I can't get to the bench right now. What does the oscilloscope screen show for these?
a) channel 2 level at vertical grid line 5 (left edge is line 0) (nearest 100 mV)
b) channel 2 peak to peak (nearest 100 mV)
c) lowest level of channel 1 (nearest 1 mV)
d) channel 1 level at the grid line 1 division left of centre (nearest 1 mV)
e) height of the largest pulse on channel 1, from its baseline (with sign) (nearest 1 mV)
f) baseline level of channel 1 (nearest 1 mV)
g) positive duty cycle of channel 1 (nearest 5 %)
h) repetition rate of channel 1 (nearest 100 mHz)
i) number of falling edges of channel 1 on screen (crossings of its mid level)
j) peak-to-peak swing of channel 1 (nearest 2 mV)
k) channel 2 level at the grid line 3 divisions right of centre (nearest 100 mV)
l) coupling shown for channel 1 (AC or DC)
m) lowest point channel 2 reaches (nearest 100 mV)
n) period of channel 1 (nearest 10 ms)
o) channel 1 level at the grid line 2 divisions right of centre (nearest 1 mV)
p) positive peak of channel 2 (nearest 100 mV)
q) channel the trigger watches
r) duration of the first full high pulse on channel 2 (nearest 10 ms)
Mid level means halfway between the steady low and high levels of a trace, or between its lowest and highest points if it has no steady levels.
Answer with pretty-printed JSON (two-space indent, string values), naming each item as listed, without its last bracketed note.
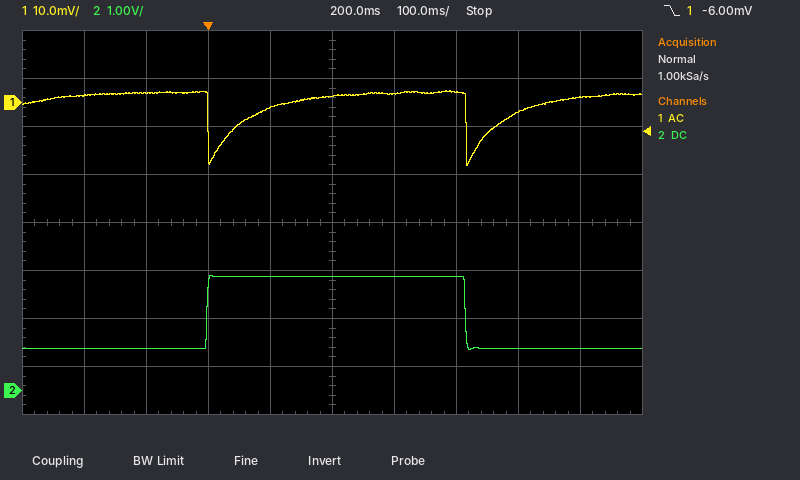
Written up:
{
  "channel 2 level at vertical grid line 5 (left edge is line 0)": "2.4 V",
  "channel 2 peak to peak": "1.5 V",
  "lowest level of channel 1": "-13 mV",
  "channel 1 level at the grid line 1 division left of centre": "-1 mV",
  "height of the largest pulse on channel 1, from its baseline (with sign)": "-15 mV",
  "baseline level of channel 1": "2 mV",
  "positive duty cycle of channel 1": "90 %",
  "repetition rate of channel 1": "2.4 Hz",
  "number of falling edges of channel 1 on screen": "2",
  "peak-to-peak swing of channel 1": "16 mV",
  "channel 2 level at the grid line 3 divisions right of centre": "900 mV",
  "coupling shown for channel 1": "AC",
  "lowest point channel 2 reaches": "900 mV",
  "period of channel 1": "420 ms",
  "channel 1 level at the grid line 2 divisions right of centre": "2 mV",
  "positive peak of channel 2": "2.4 V",
  "channel the trigger watches": "channel 1",
  "duration of the first full high pulse on channel 2": "420 ms"
}
